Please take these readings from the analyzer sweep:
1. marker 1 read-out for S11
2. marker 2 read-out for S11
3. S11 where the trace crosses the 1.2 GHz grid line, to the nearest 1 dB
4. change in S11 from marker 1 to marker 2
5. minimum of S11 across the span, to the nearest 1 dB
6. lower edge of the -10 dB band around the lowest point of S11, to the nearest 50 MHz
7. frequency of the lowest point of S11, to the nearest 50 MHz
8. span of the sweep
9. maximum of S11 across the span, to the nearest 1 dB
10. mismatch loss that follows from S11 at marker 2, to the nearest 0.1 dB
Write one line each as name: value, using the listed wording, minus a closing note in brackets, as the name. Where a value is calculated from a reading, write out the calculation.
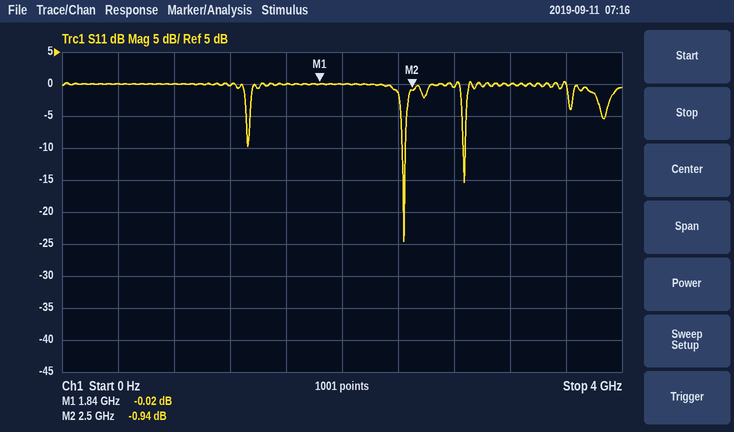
marker 1 read-out for S11: -0.02 dB
marker 2 read-out for S11: -0.94 dB
S11 where the trace crosses the 1.2 GHz grid line, to the nearest 1 dB: 0 dB
change in S11 from marker 1 to marker 2: -0.94 − (-0.02) = -0.92 dB
minimum of S11 across the span, to the nearest 1 dB: -25 dB
lower edge of the -10 dB band around the lowest point of S11, to the nearest 50 MHz: 2.45 GHz
frequency of the lowest point of S11, to the nearest 50 MHz: 2.45 GHz
span of the sweep: 4 GHz
maximum of S11 across the span, to the nearest 1 dB: 0 dB
mismatch loss that follows from S11 at marker 2, to the nearest 0.1 dB: −10 log10(1 − 10^(-0.94/10)) ≈ 7.1 dB
